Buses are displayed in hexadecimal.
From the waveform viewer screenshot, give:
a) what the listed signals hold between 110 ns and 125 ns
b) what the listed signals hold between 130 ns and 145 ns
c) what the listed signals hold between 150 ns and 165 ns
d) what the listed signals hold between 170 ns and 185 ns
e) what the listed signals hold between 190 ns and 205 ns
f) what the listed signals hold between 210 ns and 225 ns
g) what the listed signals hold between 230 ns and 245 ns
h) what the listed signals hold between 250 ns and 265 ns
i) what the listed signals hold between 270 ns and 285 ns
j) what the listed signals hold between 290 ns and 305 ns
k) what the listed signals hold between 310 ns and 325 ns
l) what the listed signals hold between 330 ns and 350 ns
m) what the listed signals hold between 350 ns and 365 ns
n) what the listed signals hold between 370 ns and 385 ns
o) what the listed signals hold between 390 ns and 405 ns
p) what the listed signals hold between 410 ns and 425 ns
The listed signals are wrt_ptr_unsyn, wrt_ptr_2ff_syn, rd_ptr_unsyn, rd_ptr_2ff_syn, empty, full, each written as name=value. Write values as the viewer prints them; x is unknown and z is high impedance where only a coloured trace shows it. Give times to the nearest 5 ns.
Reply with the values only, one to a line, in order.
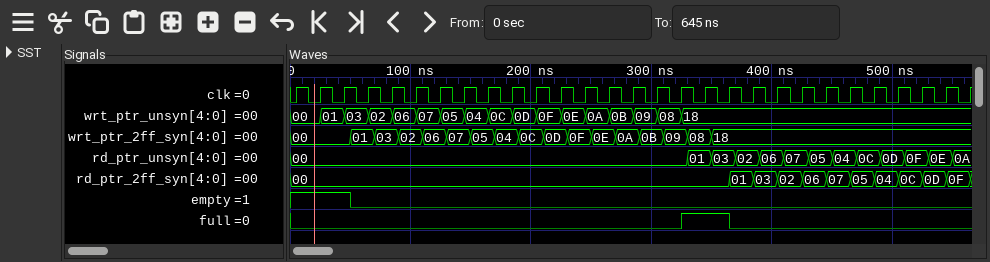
wrt_ptr_unsyn=07, wrt_ptr_2ff_syn=06, rd_ptr_unsyn=00, rd_ptr_2ff_syn=00, empty=0, full=0
wrt_ptr_unsyn=05, wrt_ptr_2ff_syn=07, rd_ptr_unsyn=00, rd_ptr_2ff_syn=00, empty=0, full=0
wrt_ptr_unsyn=04, wrt_ptr_2ff_syn=05, rd_ptr_unsyn=00, rd_ptr_2ff_syn=00, empty=0, full=0
wrt_ptr_unsyn=0C, wrt_ptr_2ff_syn=04, rd_ptr_unsyn=00, rd_ptr_2ff_syn=00, empty=0, full=0
wrt_ptr_unsyn=0D, wrt_ptr_2ff_syn=0C, rd_ptr_unsyn=00, rd_ptr_2ff_syn=00, empty=0, full=0
wrt_ptr_unsyn=0F, wrt_ptr_2ff_syn=0D, rd_ptr_unsyn=00, rd_ptr_2ff_syn=00, empty=0, full=0
wrt_ptr_unsyn=0E, wrt_ptr_2ff_syn=0F, rd_ptr_unsyn=00, rd_ptr_2ff_syn=00, empty=0, full=0
wrt_ptr_unsyn=0A, wrt_ptr_2ff_syn=0E, rd_ptr_unsyn=00, rd_ptr_2ff_syn=00, empty=0, full=0
wrt_ptr_unsyn=0B, wrt_ptr_2ff_syn=0A, rd_ptr_unsyn=00, rd_ptr_2ff_syn=00, empty=0, full=0
wrt_ptr_unsyn=09, wrt_ptr_2ff_syn=0B, rd_ptr_unsyn=00, rd_ptr_2ff_syn=00, empty=0, full=0
wrt_ptr_unsyn=08, wrt_ptr_2ff_syn=09, rd_ptr_unsyn=00, rd_ptr_2ff_syn=00, empty=0, full=0
wrt_ptr_unsyn=18, wrt_ptr_2ff_syn=08, rd_ptr_unsyn=01, rd_ptr_2ff_syn=00, empty=0, full=1
wrt_ptr_unsyn=18, wrt_ptr_2ff_syn=18, rd_ptr_unsyn=03, rd_ptr_2ff_syn=00, empty=0, full=1
wrt_ptr_unsyn=18, wrt_ptr_2ff_syn=18, rd_ptr_unsyn=02, rd_ptr_2ff_syn=01, empty=0, full=0
wrt_ptr_unsyn=18, wrt_ptr_2ff_syn=18, rd_ptr_unsyn=06, rd_ptr_2ff_syn=03, empty=0, full=0
wrt_ptr_unsyn=18, wrt_ptr_2ff_syn=18, rd_ptr_unsyn=07, rd_ptr_2ff_syn=02, empty=0, full=0
